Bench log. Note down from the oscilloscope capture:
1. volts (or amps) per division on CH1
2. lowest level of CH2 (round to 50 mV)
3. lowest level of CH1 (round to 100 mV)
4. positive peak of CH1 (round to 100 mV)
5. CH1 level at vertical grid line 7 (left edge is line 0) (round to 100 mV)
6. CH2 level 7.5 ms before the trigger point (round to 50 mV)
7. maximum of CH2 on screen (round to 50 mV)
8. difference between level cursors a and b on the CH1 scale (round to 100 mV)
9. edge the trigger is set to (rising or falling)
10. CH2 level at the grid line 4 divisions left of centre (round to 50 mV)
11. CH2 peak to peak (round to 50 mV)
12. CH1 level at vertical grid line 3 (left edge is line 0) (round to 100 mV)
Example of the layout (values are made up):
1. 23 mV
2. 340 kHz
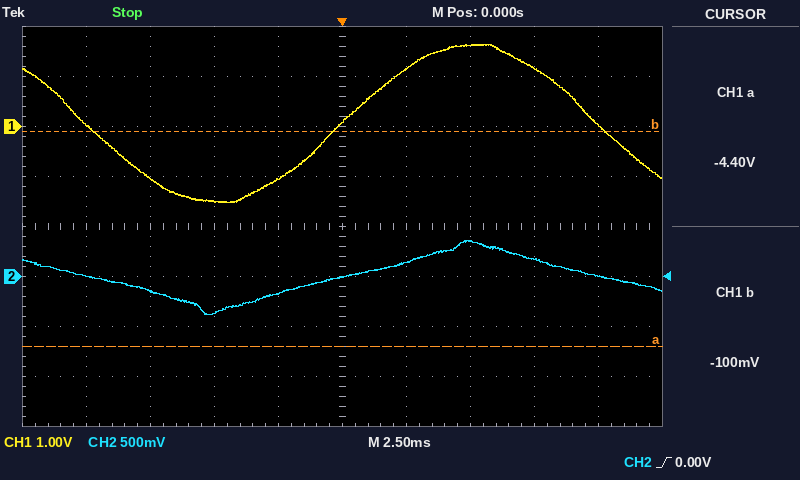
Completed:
1. 1 V
2. -400 mV
3. -1.5 V
4. 1.6 V
5. 1.6 V
6. -150 mV
7. 350 mV
8. 4.3 V
9. rising
10. 0 mV
11. 750 mV
12. -1.5 V
